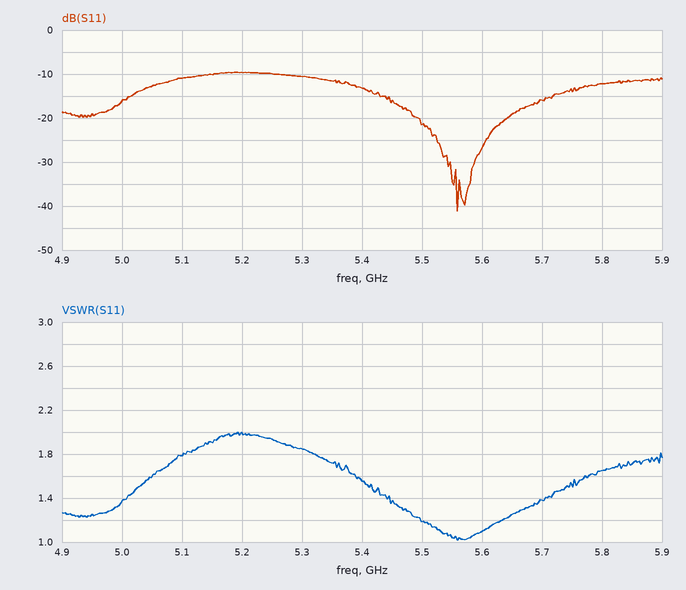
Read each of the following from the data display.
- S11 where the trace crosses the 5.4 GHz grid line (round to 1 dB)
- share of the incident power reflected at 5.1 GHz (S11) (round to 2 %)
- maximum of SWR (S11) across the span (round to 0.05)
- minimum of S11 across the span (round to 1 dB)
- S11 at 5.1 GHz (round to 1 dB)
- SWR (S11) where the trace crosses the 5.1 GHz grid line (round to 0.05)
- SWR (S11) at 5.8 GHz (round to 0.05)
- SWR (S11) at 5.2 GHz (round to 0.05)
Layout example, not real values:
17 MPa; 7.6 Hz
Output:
-13 dB; 8 %; 2.00; -41 dB; -11 dB; 1.80; 1.65; 2.00
